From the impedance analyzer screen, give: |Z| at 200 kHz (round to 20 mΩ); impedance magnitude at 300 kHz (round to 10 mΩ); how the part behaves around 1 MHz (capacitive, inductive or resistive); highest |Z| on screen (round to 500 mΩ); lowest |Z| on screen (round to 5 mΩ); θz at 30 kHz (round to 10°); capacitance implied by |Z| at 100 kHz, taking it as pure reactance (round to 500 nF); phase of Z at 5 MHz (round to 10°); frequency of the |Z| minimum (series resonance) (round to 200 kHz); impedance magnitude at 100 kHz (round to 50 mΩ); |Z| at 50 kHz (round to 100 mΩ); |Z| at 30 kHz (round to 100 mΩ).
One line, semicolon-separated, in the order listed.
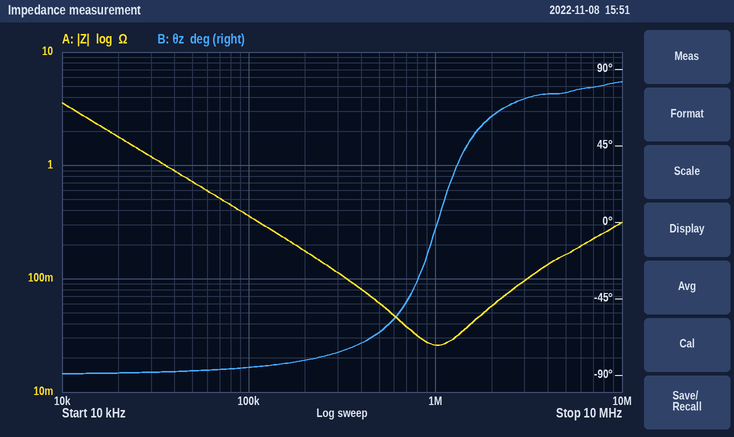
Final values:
180 mΩ; 110 mΩ; resistive; 3.5 Ω; 25 mΩ; -90°; 4.5 µF; 80°; 1.0 MHz; 350 mΩ; 700 mΩ; 1.2 Ω
